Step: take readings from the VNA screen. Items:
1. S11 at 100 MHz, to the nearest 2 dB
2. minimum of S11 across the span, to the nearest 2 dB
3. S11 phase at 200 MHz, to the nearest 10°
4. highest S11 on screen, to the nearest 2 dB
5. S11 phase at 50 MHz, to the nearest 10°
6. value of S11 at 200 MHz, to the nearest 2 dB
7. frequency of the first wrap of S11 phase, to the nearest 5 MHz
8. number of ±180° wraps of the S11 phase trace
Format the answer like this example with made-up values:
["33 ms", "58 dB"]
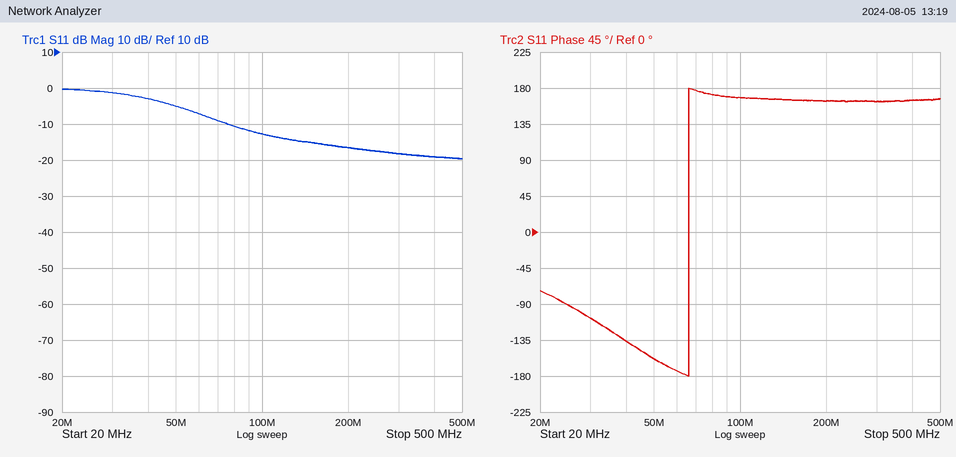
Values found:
["-12 dB", "-20 dB", "160°", "0 dB", "-160°", "-16 dB", "65 MHz", "1"]
